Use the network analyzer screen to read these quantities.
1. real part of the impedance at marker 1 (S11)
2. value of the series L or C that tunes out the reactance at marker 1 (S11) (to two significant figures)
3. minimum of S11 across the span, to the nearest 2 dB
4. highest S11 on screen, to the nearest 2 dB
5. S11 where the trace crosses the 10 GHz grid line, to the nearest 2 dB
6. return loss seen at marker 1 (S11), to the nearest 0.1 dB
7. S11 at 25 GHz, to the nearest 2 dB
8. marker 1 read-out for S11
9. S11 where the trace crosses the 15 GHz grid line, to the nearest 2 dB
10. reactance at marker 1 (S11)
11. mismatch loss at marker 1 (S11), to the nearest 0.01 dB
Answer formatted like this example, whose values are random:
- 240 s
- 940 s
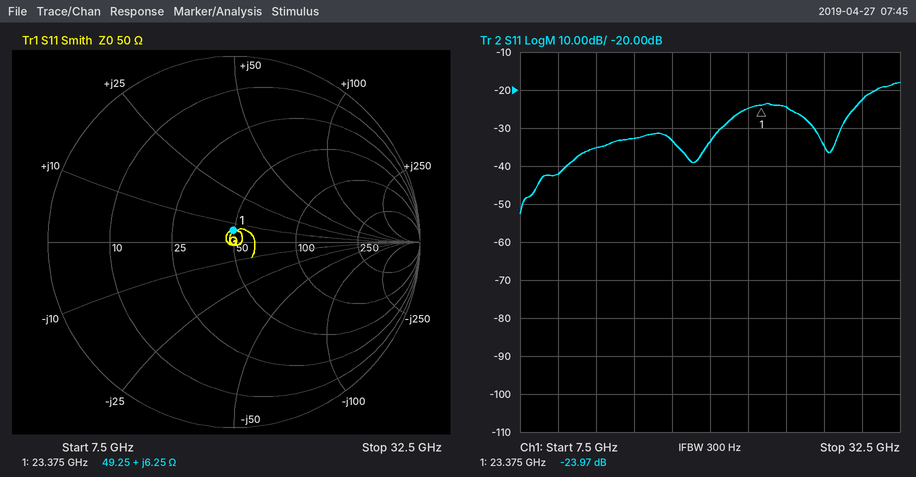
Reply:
- 49.25 Ω
- 1.1 pF
- -52 dB
- -18 dB
- -42 dB
- 24.0 dB
- -24 dB
- -23.97 dB
- -32 dB
- +6.25 Ω
- 0.02 dB
